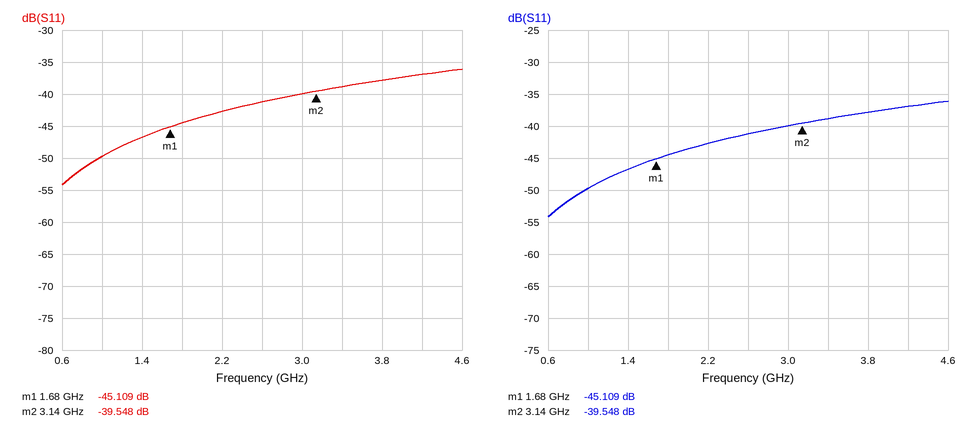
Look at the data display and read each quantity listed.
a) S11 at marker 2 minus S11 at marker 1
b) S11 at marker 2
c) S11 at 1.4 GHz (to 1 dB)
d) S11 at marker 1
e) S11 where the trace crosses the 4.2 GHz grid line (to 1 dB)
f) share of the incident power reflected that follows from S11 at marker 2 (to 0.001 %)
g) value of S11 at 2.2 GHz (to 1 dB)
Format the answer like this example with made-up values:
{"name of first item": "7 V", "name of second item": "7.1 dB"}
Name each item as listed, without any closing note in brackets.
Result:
{"S11 at marker 2 minus S11 at marker 1": "5.561 dB", "S11 at marker 2": "-39.548 dB", "S11 at 1.4 GHz": "-47 dB", "S11 at marker 1": "-45.109 dB", "S11 where the trace crosses the 4.2 GHz grid line": "-37 dB", "share of the incident power reflected that follows from S11 at marker 2": "0.011 %", "value of S11 at 2.2 GHz": "-43 dB"}
